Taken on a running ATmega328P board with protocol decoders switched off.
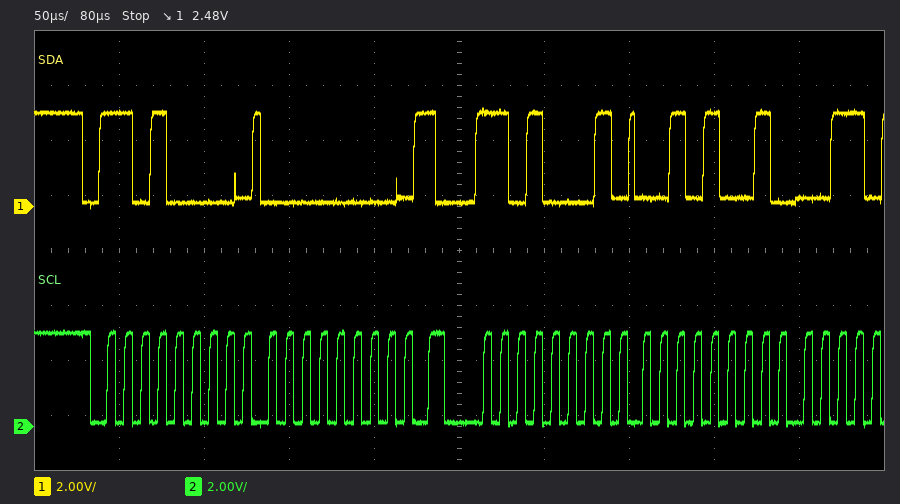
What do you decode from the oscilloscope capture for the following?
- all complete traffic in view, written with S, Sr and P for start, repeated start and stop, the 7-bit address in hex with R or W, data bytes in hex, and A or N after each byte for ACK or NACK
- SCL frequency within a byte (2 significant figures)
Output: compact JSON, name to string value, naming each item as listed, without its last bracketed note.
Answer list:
{"all complete traffic in view, written with S, Sr and P for start, repeated start and stop, the 7-bit address in hex with R or W, data bytes in hex, and A or N after each byte for ACK or NACK": "S 68W A 00 A Sr 68R A 29 A", "SCL frequency within a byte": "100 kHz"}
